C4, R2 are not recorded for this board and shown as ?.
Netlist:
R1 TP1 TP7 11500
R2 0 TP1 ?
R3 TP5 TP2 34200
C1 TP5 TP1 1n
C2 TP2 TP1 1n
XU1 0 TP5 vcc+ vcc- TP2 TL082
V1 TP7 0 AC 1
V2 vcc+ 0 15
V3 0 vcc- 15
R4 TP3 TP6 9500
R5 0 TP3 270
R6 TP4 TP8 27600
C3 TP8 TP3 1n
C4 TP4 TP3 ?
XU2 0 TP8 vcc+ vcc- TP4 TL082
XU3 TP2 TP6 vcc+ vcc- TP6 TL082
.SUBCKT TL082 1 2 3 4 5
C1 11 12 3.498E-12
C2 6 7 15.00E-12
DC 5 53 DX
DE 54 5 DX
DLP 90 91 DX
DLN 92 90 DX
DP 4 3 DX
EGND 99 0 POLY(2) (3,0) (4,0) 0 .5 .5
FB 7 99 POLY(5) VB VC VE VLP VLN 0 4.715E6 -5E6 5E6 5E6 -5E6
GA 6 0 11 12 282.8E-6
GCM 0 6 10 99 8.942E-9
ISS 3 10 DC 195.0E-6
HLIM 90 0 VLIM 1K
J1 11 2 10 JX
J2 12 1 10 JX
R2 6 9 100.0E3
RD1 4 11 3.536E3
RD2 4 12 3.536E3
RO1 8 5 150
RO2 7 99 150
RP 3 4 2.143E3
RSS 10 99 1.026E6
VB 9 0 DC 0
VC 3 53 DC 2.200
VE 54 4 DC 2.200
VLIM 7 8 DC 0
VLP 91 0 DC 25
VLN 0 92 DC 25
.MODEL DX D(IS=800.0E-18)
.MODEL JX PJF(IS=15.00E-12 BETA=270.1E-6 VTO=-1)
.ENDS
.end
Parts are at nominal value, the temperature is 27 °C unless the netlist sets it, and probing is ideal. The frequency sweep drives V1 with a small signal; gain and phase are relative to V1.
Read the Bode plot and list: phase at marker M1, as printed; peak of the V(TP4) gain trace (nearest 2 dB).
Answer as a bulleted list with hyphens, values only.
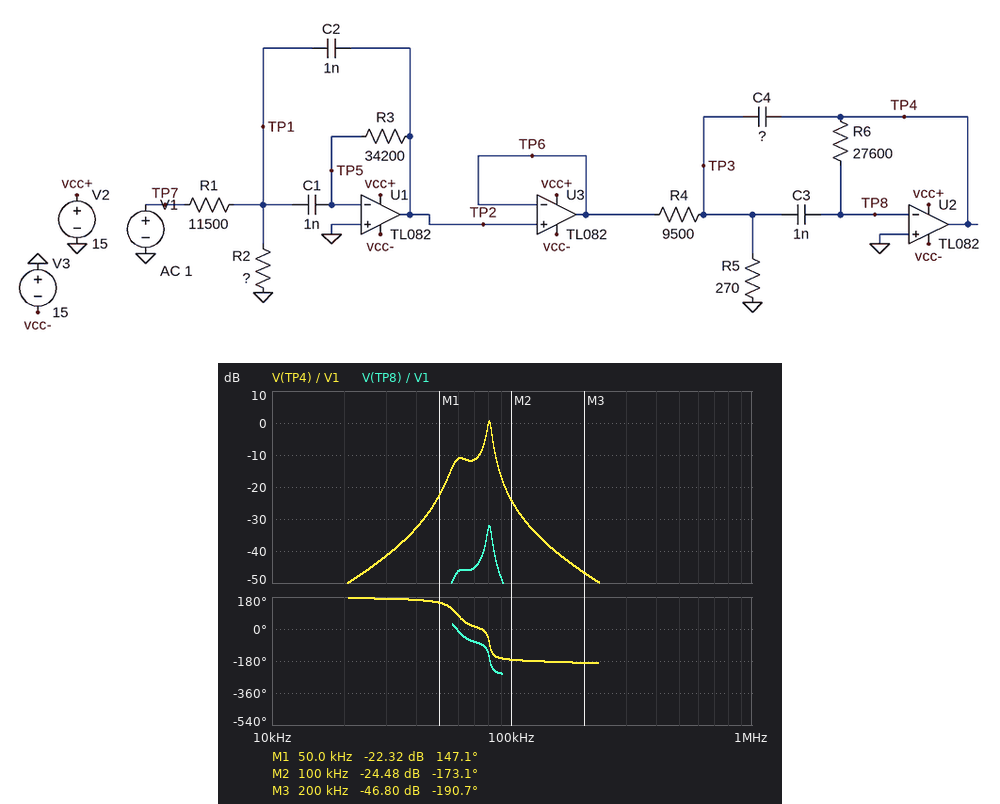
- 147.1 deg
- 0 dB
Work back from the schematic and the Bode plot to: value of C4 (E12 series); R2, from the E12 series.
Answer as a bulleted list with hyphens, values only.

- 820 pF
- 68 Ω
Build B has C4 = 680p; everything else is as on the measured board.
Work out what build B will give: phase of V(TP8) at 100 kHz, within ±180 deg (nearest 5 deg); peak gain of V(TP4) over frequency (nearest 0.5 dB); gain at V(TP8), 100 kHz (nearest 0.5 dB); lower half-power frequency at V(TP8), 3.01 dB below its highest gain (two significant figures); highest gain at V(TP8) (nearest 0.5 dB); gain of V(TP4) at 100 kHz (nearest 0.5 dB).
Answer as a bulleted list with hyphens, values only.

- 105 deg
- 3.5 dB
- -53.0 dB
- 79 kHz
- -29.0 dB
- -22.5 dB
